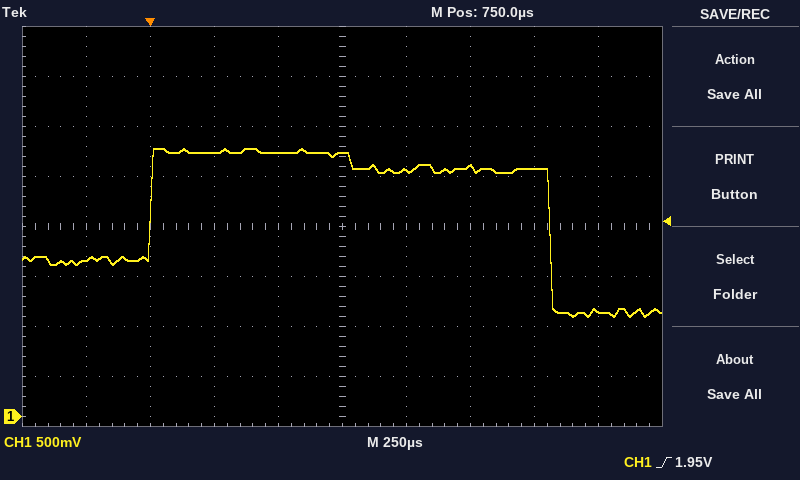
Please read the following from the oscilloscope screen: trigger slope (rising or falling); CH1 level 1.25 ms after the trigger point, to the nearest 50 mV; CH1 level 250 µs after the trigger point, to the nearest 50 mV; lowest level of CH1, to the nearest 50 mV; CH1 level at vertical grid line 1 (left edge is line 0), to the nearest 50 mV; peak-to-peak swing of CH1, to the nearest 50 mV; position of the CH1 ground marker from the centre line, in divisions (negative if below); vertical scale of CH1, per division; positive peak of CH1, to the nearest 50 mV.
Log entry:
rising
2.50 V
2.65 V
1.00 V
1.55 V
1.70 V
-3.8 div
500 mV
2.70 V
